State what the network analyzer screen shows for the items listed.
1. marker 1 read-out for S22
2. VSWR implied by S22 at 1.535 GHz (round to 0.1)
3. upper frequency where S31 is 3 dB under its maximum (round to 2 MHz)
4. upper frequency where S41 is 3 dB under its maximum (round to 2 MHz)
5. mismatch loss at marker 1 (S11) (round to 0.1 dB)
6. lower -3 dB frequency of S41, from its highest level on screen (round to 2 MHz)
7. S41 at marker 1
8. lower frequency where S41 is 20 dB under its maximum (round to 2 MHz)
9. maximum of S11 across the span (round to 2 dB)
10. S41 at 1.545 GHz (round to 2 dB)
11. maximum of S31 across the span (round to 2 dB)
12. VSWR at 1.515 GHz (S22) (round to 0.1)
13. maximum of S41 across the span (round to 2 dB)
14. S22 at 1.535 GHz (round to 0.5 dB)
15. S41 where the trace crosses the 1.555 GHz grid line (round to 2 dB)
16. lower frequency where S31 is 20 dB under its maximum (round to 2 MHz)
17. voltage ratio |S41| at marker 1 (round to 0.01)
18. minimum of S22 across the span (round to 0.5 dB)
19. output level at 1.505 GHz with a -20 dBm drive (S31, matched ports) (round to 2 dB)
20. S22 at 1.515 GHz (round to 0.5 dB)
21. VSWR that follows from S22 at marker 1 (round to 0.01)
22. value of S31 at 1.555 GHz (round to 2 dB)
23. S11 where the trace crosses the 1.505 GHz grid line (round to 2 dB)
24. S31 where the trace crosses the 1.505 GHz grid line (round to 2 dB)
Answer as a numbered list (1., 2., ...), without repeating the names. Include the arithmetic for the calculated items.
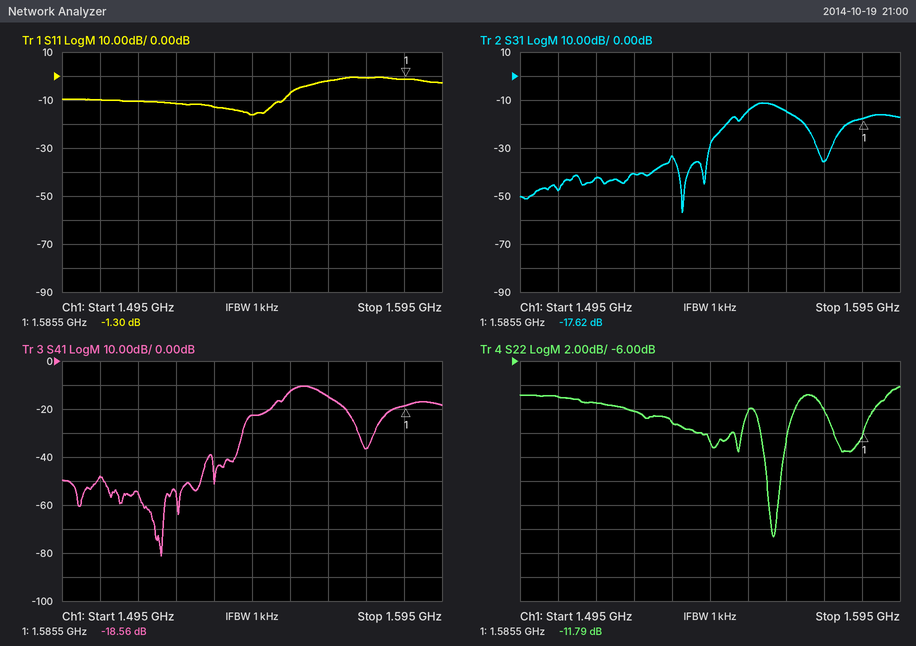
1. -11.79 dB
2. |Γ| = 10^(-11/20) = 0.2818; VSWR = (1 + 0.2818)/(1 − 0.2818) ≈ 1.8
3. 1.564 GHz
4. 1.564 GHz
5. −10 log10(1 − 10^(-1.3/10)) ≈ 5.9 dB
6. 1.554 GHz
7. -18.56 dB
8. 1.542 GHz
9. 0 dB
10. -22 dB
11. -12 dB
12. |Γ| = 10^(-9.5/20) = 0.3350; VSWR = (1 + 0.3350)/(1 − 0.3350) ≈ 2.0
13. -10 dB
14. -11.0 dB
15. -12 dB
16. 1.544 GHz
17. 10^(-18.56/20) ≈ 0.12
18. -20.5 dB
19. -20 dBm + (-48 dB) = -68 dBm
20. -9.5 dB
21. (1 + 0.2573)/(1 − 0.2573) ≈ 1.69
22. -14 dB
23. -10 dB
24. -48 dB
